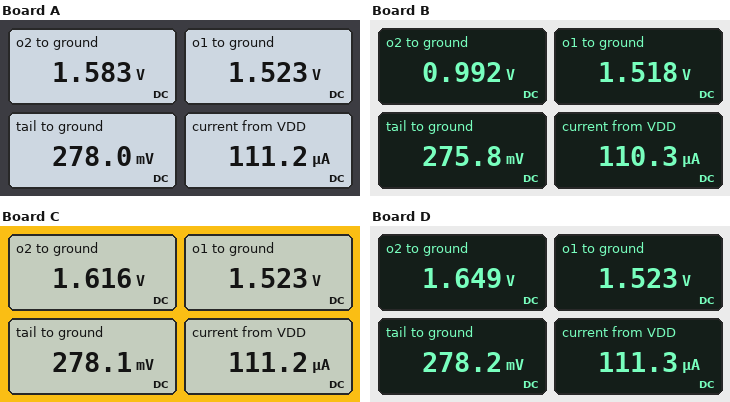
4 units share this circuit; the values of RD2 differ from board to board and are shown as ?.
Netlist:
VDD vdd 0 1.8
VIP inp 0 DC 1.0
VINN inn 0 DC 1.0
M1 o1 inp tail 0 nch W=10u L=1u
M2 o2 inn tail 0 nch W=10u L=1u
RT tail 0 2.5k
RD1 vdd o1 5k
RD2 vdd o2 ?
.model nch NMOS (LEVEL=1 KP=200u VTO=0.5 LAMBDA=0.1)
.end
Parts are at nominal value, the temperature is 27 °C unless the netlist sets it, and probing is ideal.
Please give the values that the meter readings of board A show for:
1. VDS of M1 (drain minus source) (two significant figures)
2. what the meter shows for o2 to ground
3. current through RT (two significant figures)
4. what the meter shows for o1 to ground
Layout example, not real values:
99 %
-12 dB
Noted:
1.2 V
1.583 V
110 µA
1.523 V
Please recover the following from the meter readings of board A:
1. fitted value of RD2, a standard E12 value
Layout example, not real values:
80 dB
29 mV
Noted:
3.9 kΩ
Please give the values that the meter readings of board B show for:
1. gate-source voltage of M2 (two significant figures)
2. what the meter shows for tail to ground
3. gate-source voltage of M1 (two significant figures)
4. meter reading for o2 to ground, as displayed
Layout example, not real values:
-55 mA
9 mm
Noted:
720 mV
275.8 mV
720 mV
0.992 V
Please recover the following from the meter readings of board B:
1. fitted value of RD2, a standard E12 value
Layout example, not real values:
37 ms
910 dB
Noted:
15 kΩ
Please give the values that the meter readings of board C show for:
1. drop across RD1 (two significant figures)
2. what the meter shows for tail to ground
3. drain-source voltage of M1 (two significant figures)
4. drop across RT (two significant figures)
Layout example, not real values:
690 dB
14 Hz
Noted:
280 mV
278.1 mV
1.2 V
280 mV
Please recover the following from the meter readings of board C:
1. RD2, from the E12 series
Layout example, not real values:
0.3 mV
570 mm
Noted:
3.3 kΩ
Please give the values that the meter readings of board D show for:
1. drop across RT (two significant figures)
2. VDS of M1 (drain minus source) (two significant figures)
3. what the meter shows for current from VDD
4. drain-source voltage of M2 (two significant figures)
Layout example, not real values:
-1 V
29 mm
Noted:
280 mV
1.2 V
111.3 µA
1.4 V
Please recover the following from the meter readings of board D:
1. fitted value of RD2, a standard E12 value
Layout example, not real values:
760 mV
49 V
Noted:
2.7 kΩ
